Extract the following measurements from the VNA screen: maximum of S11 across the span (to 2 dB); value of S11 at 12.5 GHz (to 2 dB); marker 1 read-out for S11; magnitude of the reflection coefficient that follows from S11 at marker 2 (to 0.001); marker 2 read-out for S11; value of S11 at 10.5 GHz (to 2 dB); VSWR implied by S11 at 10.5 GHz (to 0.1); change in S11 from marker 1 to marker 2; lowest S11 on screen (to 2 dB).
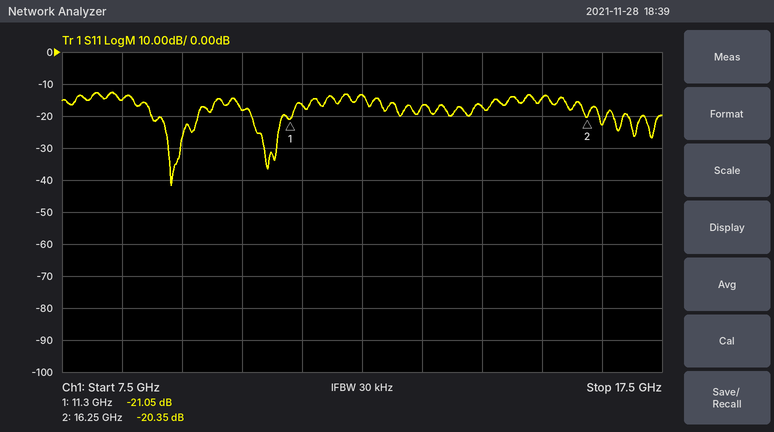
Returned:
-12 dB
-14 dB
-21.05 dB
0.096
-20.35 dB
-18 dB
1.3
0.70 dB
-42 dB
